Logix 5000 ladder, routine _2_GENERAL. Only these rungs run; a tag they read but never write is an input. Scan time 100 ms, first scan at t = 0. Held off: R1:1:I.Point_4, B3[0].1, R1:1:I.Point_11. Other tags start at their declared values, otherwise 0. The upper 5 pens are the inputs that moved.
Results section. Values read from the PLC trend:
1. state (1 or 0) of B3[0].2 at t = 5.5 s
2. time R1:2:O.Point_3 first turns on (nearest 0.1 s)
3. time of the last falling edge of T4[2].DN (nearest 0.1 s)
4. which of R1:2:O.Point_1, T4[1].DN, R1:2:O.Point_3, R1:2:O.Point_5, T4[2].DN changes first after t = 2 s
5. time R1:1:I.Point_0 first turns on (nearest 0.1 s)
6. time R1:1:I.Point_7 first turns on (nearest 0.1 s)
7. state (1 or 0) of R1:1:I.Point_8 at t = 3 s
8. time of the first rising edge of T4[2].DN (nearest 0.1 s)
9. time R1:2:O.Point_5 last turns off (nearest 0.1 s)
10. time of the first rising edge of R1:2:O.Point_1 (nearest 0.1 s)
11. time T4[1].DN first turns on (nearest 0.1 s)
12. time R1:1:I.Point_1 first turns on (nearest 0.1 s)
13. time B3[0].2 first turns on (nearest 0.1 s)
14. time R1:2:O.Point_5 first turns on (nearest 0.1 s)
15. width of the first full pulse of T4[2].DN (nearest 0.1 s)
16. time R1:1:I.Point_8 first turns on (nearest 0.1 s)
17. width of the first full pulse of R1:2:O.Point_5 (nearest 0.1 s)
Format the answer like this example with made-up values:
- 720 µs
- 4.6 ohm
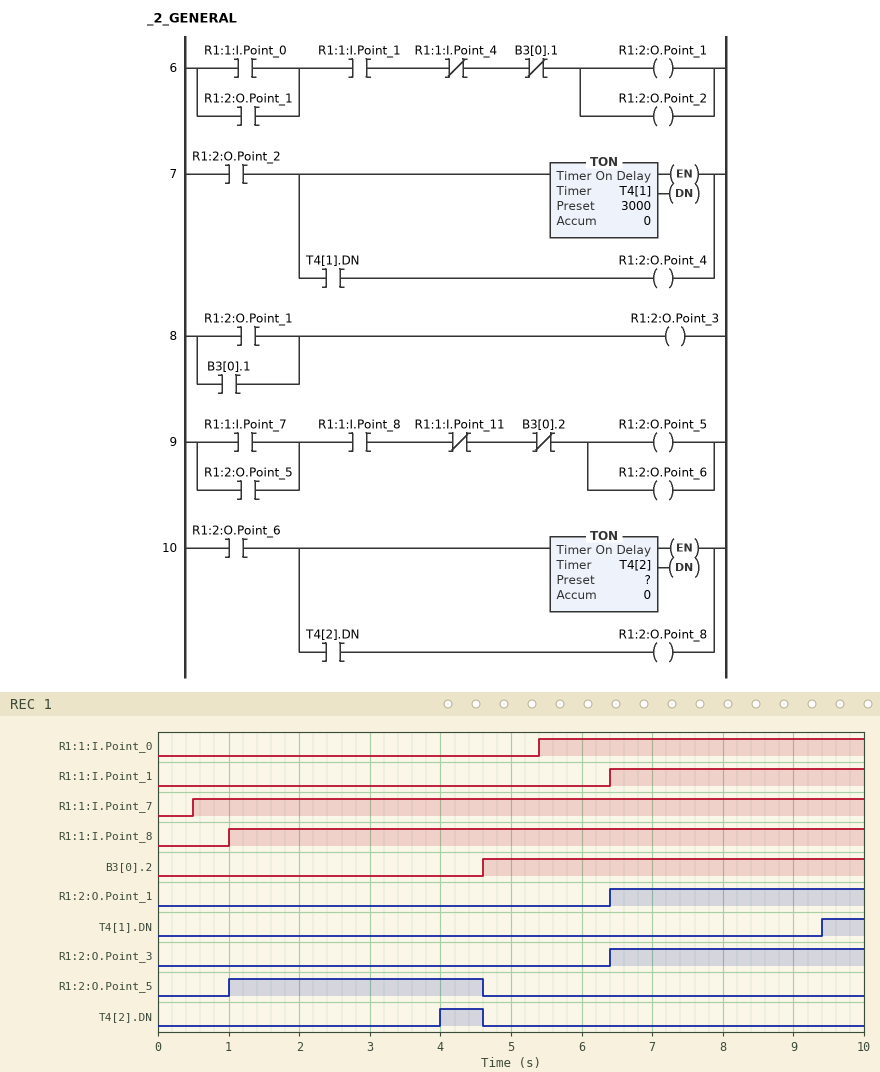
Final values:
- 1
- 6.4 s
- 4.6 s
- T4[2].DN
- 5.4 s
- 0.5 s
- 1
- 4.0 s
- 4.6 s
- 6.4 s
- 9.4 s
- 6.4 s
- 4.6 s
- 1.0 s
- 0.6 s
- 1.0 s
- 3.6 s
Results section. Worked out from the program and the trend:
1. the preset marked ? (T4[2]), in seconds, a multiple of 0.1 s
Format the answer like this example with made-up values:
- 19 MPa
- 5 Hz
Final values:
- 3.0 s
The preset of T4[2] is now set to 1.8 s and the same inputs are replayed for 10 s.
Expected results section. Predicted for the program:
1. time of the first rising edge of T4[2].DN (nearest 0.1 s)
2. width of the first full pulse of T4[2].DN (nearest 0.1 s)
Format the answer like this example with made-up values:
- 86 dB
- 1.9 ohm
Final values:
- 2.8 s
- 1.8 s
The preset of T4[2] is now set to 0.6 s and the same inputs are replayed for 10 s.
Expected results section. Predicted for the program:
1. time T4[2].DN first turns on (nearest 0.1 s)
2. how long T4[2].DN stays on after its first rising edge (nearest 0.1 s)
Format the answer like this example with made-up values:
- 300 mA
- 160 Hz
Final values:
- 1.6 s
- 3.0 s
